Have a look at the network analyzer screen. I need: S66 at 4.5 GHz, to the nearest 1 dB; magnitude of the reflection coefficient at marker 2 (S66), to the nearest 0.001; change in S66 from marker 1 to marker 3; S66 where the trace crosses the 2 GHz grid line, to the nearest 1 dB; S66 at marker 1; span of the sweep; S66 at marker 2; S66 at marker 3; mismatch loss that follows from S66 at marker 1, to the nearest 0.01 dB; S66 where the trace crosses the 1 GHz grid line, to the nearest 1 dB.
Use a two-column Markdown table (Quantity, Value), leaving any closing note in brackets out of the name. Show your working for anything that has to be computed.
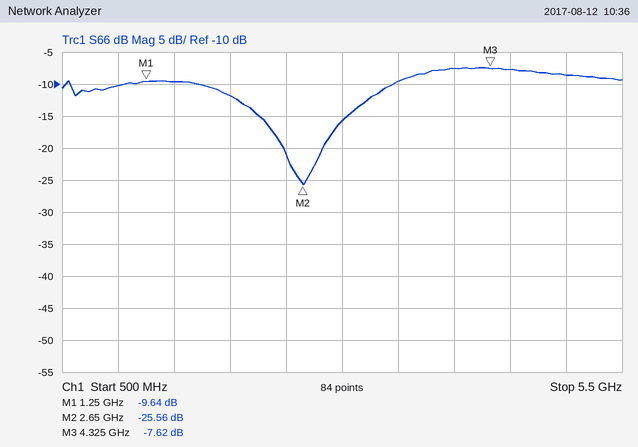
| Quantity | Value |
|---|---|
| S66 at 4.5 GHz, to the nearest 1 dB | -8 dB |
| magnitude of the reflection coefficient at marker 2 (S66), to the nearest 0.001 | 10^(-25.56/20) ≈ 0.053 |
| change in S66 from marker 1 to marker 3 | -7.62 − (-9.64) = 2.02 dB |
| S66 where the trace crosses the 2 GHz grid line, to the nearest 1 dB | -12 dB |
| S66 at marker 1 | -9.64 dB |
| span of the sweep | 5 GHz |
| S66 at marker 2 | -25.56 dB |
| S66 at marker 3 | -7.62 dB |
| mismatch loss that follows from S66 at marker 1, to the nearest 0.01 dB | −10 log10(1 − 10^(-9.64/10)) ≈ 0.50 dB |
| S66 where the trace crosses the 1 GHz grid line, to the nearest 1 dB | -10 dB |
